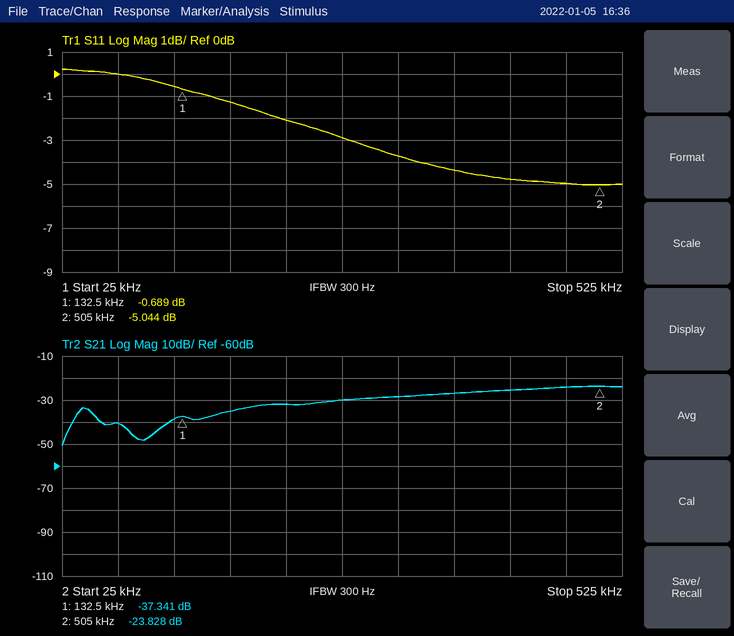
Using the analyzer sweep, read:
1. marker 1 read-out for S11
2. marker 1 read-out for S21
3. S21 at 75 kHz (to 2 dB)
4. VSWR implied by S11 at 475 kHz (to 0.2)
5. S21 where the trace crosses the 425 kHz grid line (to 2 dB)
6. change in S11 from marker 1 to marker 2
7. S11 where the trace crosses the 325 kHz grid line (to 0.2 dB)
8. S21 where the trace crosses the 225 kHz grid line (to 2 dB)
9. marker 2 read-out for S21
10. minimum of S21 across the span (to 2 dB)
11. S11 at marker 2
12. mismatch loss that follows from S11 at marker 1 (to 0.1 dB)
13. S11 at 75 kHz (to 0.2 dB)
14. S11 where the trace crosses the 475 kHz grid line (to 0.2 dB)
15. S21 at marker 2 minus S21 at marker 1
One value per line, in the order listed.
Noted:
-0.689 dB
-37.341 dB
-40 dB
3.6
-26 dB
-4.355 dB
-3.8 dB
-32 dB
-23.828 dB
-50 dB
-5.044 dB
8.3 dB
0.0 dB
-5.0 dB
13.513 dB
